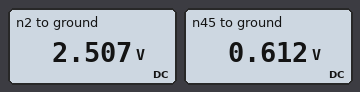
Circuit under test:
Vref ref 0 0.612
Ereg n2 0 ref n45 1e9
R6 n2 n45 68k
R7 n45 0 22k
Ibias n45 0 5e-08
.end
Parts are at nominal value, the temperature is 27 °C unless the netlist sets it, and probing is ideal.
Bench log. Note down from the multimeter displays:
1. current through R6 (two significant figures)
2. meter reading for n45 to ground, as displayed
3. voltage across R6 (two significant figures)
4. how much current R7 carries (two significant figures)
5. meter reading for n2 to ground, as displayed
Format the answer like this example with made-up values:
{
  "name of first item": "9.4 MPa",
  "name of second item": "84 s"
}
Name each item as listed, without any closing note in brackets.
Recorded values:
{
  "current through R6": "28 µA",
  "meter reading for n45 to ground, as displayed": "0.612 V",
  "voltage across R6": "1.9 V",
  "how much current R7 carries": "28 µA",
  "meter reading for n2 to ground, as displayed": "2.507 V"
}
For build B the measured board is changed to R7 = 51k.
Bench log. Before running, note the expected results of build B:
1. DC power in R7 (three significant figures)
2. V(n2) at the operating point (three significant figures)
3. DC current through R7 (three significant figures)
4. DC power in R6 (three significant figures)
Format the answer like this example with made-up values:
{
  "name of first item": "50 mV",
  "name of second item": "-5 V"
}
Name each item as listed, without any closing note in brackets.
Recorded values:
{
  "DC power in R7": "7.34 µW",
  "V(n2) at the operating point": "1.43 V",
  "DC current through R7": "12.0 µA",
  "DC power in R6": "9.87 µW"
}
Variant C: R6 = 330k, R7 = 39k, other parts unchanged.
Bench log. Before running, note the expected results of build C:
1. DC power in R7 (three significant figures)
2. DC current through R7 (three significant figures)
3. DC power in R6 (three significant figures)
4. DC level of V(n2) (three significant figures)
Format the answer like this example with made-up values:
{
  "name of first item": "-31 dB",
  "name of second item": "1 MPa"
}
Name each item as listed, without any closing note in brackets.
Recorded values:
{
  "DC power in R7": "9.60 µW",
  "DC current through R7": "15.7 µA",
  "DC power in R6": "81.8 µW",
  "DC level of V(n2)": "5.81 V"
}
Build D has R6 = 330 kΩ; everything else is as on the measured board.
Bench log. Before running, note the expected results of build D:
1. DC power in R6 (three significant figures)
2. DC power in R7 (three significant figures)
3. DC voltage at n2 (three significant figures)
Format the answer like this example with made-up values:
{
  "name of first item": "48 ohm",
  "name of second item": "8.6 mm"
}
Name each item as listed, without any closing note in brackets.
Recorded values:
{
  "DC power in R6": "256 µW",
  "DC power in R7": "17.0 µW",
  "DC voltage at n2": "9.81 V"
}
